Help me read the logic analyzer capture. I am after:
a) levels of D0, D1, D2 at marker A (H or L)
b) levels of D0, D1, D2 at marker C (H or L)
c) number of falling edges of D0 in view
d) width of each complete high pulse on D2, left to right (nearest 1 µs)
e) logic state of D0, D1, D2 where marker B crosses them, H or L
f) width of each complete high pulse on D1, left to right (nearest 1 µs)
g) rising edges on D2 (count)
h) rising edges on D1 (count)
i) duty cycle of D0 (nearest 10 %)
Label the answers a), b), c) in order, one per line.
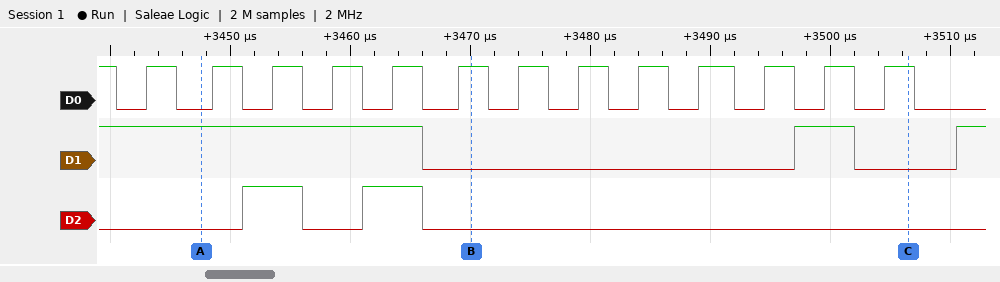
a) D0=L, D1=H, D2=L
b) D0=H, D1=L, D2=L
c) 14
d) 5 µs, 5 µs
e) D0=H, D1=L, D2=L
f) 5 µs
g) 2
h) 2
i) 50 %
